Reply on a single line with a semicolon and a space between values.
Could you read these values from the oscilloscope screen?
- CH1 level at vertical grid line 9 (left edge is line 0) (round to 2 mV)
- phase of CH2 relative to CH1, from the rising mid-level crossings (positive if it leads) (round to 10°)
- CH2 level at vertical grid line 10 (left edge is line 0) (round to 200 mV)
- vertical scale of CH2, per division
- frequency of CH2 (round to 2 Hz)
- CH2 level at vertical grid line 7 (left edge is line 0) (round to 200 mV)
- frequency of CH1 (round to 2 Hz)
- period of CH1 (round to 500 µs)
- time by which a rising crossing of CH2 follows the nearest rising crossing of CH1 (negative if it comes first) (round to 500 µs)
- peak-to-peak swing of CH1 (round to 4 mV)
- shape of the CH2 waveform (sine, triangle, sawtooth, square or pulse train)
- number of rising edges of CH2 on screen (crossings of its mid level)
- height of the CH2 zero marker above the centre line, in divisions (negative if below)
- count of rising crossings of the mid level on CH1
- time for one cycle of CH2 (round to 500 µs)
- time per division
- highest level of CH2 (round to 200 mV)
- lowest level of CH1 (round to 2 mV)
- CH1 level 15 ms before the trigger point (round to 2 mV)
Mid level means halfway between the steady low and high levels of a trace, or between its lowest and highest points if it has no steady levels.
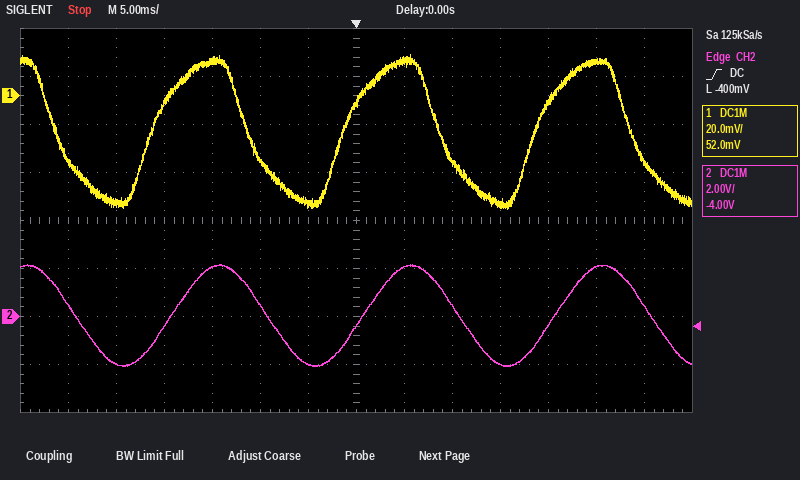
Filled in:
-28 mV; -40°; -2.0 V; 2 V; 50 Hz; -400 mV; 50 Hz; 20.0 ms; +2.0 ms; 64 mV; sine; 3; -2.0 div; 3; 20.0 ms; 5 ms; 2.2 V; -48 mV; 14 mV
